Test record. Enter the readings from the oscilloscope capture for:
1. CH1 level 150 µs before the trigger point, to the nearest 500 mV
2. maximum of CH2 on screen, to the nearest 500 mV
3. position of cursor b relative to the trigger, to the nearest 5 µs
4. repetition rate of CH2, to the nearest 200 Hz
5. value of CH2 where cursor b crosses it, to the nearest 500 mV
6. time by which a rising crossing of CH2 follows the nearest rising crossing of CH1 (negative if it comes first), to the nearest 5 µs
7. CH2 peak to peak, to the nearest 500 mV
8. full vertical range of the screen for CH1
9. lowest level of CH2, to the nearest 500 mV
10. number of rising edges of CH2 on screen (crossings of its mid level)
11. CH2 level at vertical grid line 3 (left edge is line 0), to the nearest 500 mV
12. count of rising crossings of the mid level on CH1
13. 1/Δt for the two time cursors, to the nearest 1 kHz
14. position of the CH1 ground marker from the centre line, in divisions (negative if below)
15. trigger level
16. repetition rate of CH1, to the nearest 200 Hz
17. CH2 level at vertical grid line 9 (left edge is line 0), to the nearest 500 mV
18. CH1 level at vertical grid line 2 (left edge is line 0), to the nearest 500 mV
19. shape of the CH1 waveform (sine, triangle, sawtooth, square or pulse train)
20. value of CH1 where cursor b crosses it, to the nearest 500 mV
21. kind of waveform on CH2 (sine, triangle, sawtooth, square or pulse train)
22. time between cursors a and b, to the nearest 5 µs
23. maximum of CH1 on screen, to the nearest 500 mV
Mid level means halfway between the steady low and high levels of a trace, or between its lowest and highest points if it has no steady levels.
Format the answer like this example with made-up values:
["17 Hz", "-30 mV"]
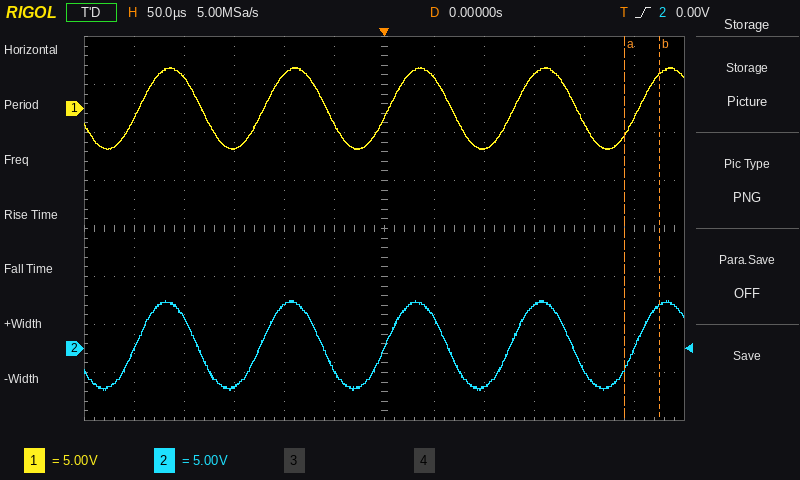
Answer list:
["-4.0 V", "5.0 V", "+275 µs", "8.0 kHz", "4.5 V", "-5 µs", "9.5 V", "40 V", "-4.5 V", "5", "-4.0 V", "5", "29 kHz", "+2.5 div", "0.00 V", "8.0 kHz", "4.5 V", "3.0 V", "sine", "3.5 V", "sine", "35 µs", "4.5 V"]
